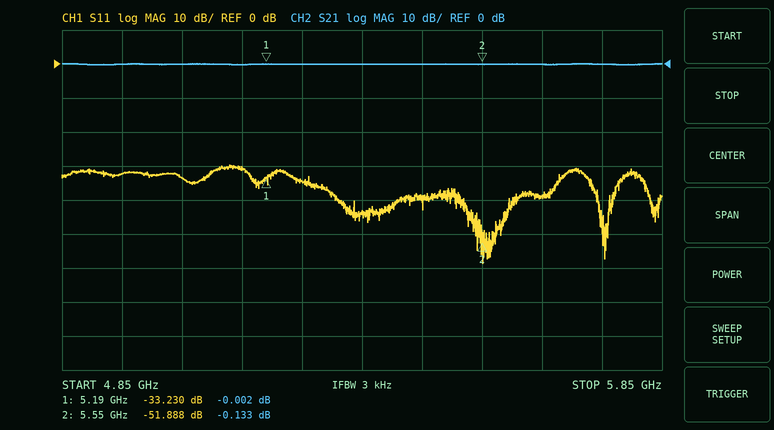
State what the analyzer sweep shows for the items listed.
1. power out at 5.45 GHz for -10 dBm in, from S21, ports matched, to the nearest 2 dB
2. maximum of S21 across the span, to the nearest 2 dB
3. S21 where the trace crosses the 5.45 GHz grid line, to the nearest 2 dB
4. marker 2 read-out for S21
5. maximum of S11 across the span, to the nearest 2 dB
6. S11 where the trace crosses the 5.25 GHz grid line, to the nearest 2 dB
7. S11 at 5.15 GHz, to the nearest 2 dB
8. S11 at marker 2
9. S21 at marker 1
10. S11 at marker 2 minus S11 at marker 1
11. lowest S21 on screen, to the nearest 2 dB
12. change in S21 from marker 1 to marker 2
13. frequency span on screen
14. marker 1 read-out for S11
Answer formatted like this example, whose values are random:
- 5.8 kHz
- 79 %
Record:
- -10 dBm
- 0 dB
- 0 dB
- -0.133 dB
- -30 dB
- -34 dB
- -30 dB
- -51.888 dB
- -0.002 dB
- -18.658 dB
- 0 dB
- -0.131 dB
- 1 GHz
- -33.230 dB
